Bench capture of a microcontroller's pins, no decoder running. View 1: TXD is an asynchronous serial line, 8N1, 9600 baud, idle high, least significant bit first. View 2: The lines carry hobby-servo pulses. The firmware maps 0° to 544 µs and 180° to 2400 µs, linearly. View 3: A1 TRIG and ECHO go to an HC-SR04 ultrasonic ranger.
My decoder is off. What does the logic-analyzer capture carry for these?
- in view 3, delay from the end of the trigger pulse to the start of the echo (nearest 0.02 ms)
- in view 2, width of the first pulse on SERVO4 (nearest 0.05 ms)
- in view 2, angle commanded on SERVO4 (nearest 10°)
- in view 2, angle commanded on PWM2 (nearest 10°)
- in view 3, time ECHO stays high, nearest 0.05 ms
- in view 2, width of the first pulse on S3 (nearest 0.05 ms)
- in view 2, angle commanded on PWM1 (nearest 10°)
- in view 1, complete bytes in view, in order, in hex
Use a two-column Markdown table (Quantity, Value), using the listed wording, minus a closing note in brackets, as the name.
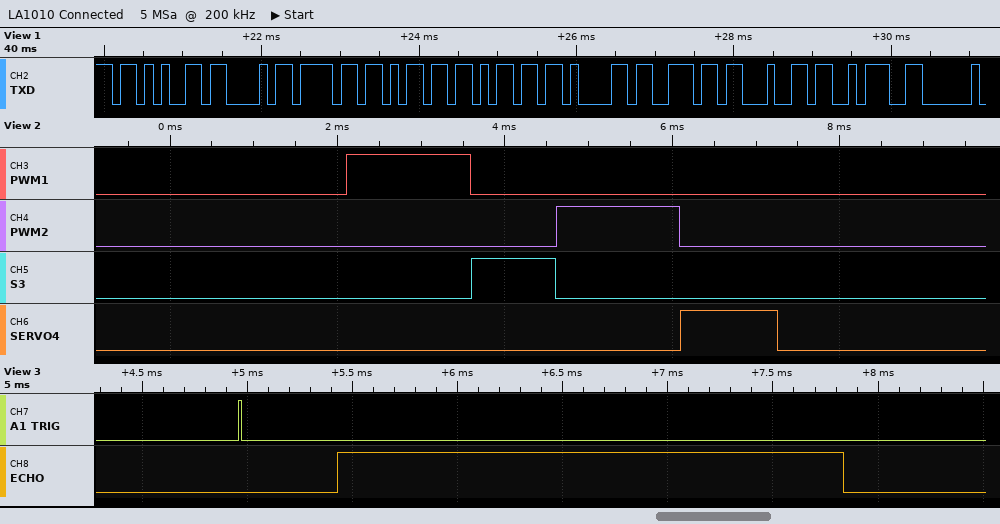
| Quantity | Value |
|---|---|
| in view 3, delay from the end of the trigger pulse to the start of the echo | 0.46 ms |
| in view 2, width of the first pulse on SERVO4 | 1.15 ms |
| in view 2, angle commanded on SERVO4 | 60° |
| in view 2, angle commanded on PWM2 | 90° |
| in view 3, time ECHO stays high, nearest 0.05 ms | 2.40 ms |
| in view 2, width of the first pulse on S3 | 1.00 ms |
| in view 2, angle commanded on PWM1 | 90° |
| in view 1, complete bytes in view, in order, in hex | 2B 43 6F 6D 6D 61 6E 64 3A |
